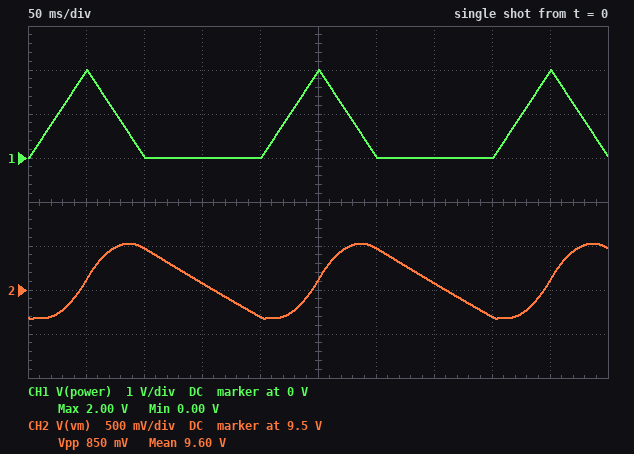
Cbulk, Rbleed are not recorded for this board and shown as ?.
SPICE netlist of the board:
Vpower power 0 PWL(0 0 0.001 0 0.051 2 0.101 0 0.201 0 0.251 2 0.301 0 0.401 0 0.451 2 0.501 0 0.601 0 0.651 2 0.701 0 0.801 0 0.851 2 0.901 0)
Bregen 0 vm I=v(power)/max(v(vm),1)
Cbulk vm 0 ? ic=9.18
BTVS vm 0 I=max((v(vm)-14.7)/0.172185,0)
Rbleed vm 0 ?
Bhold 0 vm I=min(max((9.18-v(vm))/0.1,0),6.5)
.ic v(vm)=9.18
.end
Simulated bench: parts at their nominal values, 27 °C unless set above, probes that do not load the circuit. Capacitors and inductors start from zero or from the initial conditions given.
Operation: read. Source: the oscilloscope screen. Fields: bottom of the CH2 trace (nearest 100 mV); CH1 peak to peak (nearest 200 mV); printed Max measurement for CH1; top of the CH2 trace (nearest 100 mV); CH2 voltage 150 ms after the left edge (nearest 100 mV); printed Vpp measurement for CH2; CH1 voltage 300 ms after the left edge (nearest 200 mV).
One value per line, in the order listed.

9.2 V
2.0 V
2.00 V
10.0 V
9.6 V
850 mV
0 V
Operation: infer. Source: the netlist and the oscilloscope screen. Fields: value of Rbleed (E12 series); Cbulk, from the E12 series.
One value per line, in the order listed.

180 Ω
6.8 mF
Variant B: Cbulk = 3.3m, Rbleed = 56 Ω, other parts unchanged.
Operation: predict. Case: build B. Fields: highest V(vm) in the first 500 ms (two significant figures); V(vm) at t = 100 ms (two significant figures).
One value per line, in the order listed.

9.4 V
9.2 V
